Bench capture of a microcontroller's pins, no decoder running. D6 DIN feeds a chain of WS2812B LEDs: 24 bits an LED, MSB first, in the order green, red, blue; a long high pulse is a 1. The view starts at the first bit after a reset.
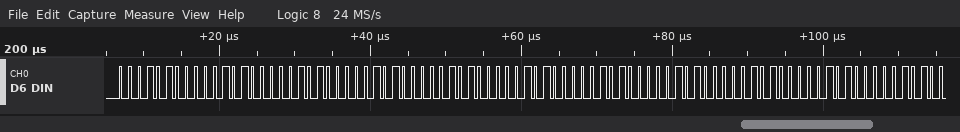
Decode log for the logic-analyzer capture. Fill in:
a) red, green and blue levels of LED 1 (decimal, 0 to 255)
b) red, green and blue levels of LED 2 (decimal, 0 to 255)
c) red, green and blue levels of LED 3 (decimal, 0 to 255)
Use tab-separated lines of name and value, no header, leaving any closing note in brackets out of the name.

red, green and blue levels of LED 1	20, 20, 20
red, green and blue levels of LED 2	20, 20, 20
red, green and blue levels of LED 3	20, 20, 20
